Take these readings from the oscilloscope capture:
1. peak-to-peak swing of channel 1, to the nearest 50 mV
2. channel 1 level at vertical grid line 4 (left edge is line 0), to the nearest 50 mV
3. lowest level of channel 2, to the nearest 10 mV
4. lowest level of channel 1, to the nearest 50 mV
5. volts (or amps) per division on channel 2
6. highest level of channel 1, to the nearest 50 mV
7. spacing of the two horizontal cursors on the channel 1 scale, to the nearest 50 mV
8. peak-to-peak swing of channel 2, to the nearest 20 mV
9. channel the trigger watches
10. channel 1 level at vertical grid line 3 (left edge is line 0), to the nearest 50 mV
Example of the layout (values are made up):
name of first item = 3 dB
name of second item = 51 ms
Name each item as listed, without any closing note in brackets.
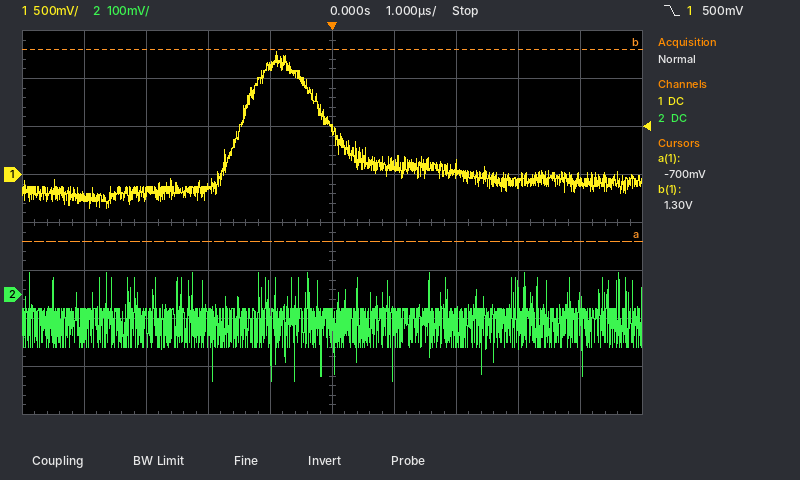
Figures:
peak-to-peak swing of channel 1, to the nearest 50 mV = 1.65 V
channel 1 level at vertical grid line 4 (left edge is line 0), to the nearest 50 mV = 1.15 V
lowest level of channel 2, to the nearest 10 mV = -180 mV
lowest level of channel 1, to the nearest 50 mV = -350 mV
volts (or amps) per division on channel 2 = 100 mV
highest level of channel 1, to the nearest 50 mV = 1.30 V
spacing of the two horizontal cursors on the channel 1 scale, to the nearest 50 mV = 2.00 V
peak-to-peak swing of channel 2, to the nearest 20 mV = 220 mV
channel the trigger watches = channel 1
channel 1 level at vertical grid line 3 (left edge is line 0), to the nearest 50 mV = -150 mV
